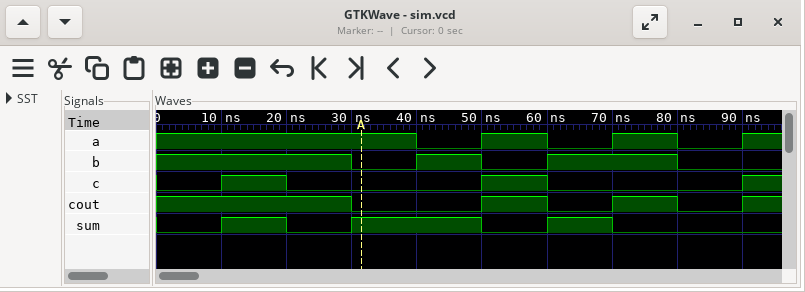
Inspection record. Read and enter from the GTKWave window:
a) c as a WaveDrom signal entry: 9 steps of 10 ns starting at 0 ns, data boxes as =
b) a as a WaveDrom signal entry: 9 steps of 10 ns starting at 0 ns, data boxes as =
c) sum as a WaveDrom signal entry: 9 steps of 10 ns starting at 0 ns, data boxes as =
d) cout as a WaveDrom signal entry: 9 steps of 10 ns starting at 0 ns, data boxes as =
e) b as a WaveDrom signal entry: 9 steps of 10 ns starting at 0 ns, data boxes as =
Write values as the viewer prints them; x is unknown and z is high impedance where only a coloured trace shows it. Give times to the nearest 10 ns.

{name: 'c', wave: '010..10..'}
{name: 'a', wave: '1...01010'}
{name: 'sum', wave: '0101.010.'}
{name: 'cout', wave: '1..0.1010'}
{name: 'b', wave: '1..0101.0'}
